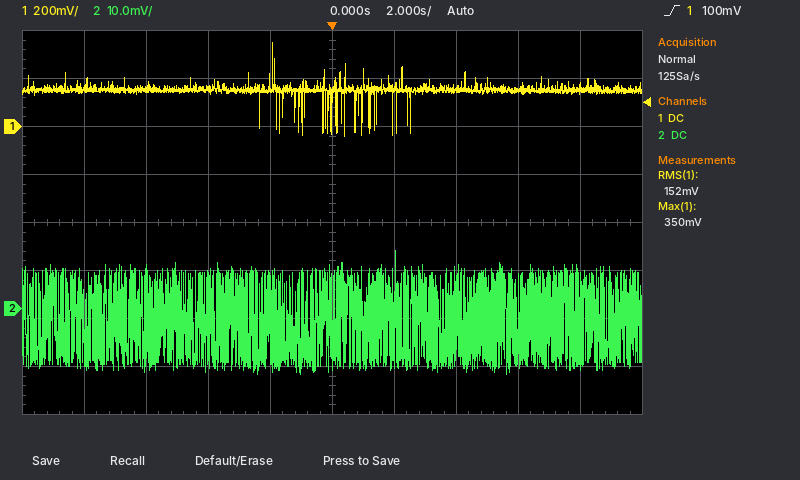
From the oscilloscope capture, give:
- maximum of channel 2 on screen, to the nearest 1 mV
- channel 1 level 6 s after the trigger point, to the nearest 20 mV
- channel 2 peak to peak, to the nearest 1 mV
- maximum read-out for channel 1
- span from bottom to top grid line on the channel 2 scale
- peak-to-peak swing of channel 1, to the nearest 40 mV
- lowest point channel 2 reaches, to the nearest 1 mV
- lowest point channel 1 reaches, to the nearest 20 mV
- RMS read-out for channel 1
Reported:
12 mV
160 mV
26 mV
350 mV
80 mV
400 mV
-14 mV
-40 mV
152 mV
